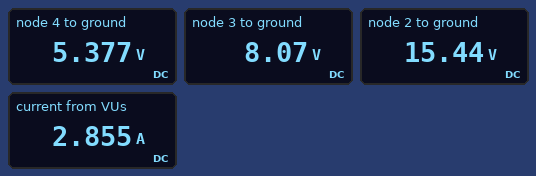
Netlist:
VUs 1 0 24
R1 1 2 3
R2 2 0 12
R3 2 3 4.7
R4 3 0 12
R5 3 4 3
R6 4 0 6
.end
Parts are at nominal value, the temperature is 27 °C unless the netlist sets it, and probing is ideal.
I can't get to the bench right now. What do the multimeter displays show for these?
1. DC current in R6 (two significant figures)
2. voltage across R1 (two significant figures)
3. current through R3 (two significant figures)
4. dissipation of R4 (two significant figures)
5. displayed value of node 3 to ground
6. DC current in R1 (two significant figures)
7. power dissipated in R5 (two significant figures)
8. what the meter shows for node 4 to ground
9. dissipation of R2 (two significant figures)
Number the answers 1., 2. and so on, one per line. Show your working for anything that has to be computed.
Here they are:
1. (5.377 V) / 6 Ω = 900 mA
2. 24 V - 15.44 V = 8.6 V
3. (15.44 V - 8.07 V) / 4.7 Ω = 1.6 A
4. (8.07 V)^2 / 12 Ω = 5.4 W
5. 8.07 V
6. (24 V - 15.44 V) / 3 Ω = 2.9 A
7. (8.07 V - 5.377 V)^2 / 3 Ω = 2.4 W
8. 5.377 V
9. (15.44 V)^2 / 12 Ω = 20 W
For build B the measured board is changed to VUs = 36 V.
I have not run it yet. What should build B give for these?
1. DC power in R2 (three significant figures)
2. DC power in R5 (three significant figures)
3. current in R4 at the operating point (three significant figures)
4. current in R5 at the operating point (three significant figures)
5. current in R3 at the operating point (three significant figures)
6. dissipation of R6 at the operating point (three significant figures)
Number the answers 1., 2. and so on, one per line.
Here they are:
1. 44.7 W
2. 5.42 W
3. 1.01 A
4. 1.34 A
5. 2.35 A
6. 10.8 W
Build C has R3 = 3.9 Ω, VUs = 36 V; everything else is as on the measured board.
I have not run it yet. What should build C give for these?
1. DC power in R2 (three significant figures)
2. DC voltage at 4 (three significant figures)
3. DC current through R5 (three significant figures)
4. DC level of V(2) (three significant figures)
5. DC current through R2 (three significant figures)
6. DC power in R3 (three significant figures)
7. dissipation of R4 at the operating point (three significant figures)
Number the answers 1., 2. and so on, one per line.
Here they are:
1. 43.2 W
2. 8.63 V
3. 1.44 A
4. 22.8 V
5. 1.90 A
6. 24.7 W
7. 14.0 W
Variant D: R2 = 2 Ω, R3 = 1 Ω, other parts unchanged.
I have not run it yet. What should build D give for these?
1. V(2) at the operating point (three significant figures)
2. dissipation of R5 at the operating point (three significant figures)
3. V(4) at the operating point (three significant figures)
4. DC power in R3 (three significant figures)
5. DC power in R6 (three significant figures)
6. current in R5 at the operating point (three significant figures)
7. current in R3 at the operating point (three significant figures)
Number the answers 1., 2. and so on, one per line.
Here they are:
1. 8.03 V
2. 1.67 W
3. 4.48 V
4. 1.71 W
5. 3.35 W
6. 747 mA
7. 1.31 A
